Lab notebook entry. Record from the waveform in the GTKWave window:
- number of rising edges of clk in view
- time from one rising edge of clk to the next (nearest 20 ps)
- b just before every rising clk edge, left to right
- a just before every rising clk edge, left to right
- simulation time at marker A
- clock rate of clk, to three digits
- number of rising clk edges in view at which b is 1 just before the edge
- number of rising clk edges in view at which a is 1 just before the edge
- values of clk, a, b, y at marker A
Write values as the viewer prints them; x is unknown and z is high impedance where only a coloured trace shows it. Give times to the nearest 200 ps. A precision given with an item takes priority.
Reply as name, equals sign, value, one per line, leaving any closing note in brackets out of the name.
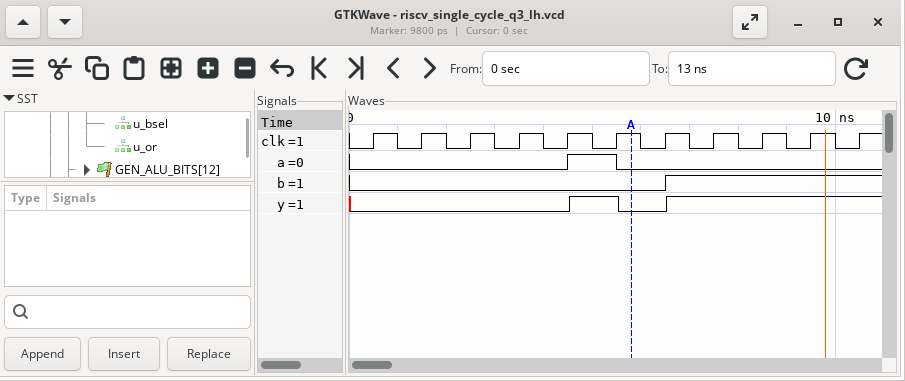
number of rising edges of clk in view = 11
time from one rising edge of clk to the next = 1000 ps
b just before every rising clk edge, left to right = 0 0 0 0 0 0 0 1 1 1 1
a just before every rising clk edge, left to right = 0 0 0 0 0 1 0 0 0 0 0
simulation time at marker A = 5800 ps
clock rate of clk, to three digits = 1.00 GHz
number of rising clk edges in view at which b is 1 just before the edge = 4
number of rising clk edges in view at which a is 1 just before the edge = 1
values of clk, a, b, y at marker A = clk=1, a=0, b=0, y=0
